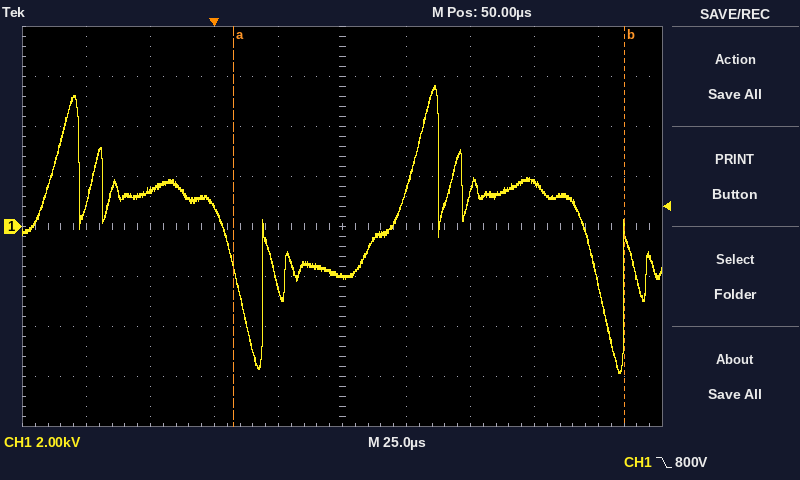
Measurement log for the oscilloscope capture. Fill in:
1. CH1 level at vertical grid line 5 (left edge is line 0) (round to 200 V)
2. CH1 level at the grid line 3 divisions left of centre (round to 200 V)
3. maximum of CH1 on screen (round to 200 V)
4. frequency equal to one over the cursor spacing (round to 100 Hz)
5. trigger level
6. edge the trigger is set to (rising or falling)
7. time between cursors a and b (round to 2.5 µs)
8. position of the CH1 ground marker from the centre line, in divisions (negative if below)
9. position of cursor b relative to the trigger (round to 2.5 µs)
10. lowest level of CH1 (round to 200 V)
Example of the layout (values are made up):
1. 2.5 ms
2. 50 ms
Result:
1. -2.0 kV
2. 1.4 kV
3. 5.6 kV
4. 6.6 kHz
5. 800 V
6. falling
7. 152.5 µs
8. 0.0 div
9. +160.0 µs
10. -5.8 kV
